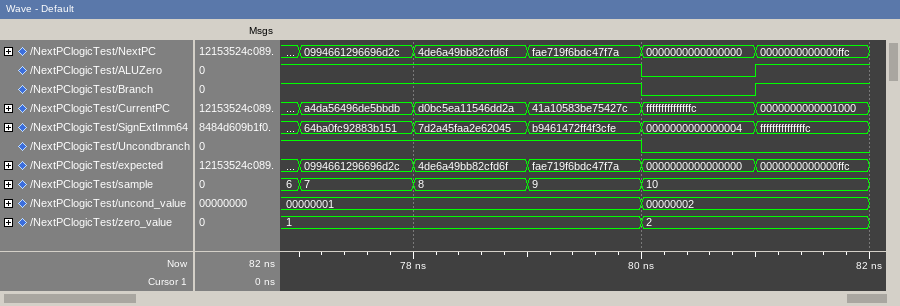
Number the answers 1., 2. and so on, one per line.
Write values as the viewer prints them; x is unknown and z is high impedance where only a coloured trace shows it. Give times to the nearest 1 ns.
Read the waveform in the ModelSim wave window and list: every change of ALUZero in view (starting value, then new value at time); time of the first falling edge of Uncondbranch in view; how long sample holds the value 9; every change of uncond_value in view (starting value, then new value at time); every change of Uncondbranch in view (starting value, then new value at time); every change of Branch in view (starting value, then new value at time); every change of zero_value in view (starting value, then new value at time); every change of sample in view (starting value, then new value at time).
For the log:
1. 1, 0 at 80 ns, 1 at 81 ns
2. 80 ns
3. 1 ns
4. 00000001, 00000002 at 80 ns
5. 1, 0 at 80 ns
6. 1, 0 at 80 ns, 1 at 81 ns
7. 1, 2 at 80 ns
8. 6, 7 at 77 ns, 8 at 78 ns, 9 at 79 ns, 10 at 80 ns
